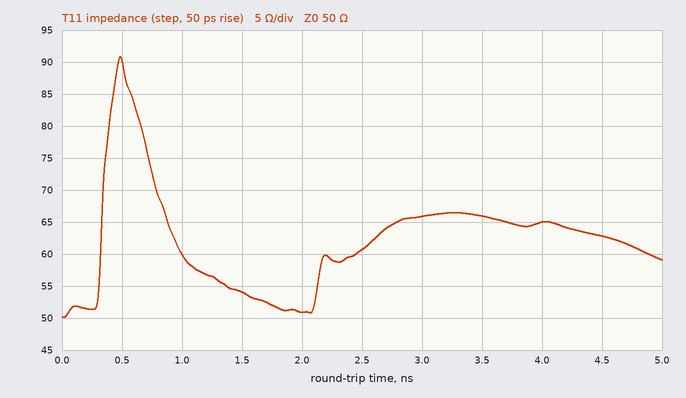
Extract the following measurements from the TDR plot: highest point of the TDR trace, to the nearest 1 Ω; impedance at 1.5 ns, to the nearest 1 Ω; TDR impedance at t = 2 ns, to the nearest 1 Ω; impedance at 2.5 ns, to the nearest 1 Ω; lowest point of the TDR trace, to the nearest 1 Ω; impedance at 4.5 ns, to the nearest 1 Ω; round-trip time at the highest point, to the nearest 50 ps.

91 Ω
54 Ω
51 Ω
61 Ω
50 Ω
63 Ω
500 ps
